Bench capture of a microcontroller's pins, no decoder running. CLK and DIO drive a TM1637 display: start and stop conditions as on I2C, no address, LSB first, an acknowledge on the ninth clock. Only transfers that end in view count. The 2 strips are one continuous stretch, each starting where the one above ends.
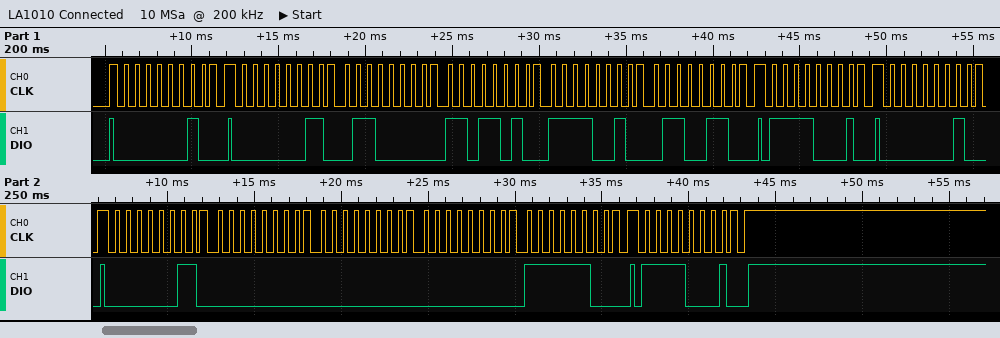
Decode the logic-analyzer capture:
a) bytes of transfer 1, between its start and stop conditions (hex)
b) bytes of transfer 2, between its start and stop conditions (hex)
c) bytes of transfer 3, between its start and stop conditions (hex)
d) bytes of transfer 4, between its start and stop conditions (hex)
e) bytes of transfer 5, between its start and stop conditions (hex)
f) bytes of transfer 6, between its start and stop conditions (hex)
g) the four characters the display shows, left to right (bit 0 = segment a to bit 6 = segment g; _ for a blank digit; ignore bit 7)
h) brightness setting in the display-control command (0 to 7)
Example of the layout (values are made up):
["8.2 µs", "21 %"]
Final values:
["40", "C0 06 5B 4F 66", "8F", "40", "C0 00 00 00 3F", "8F", "___0", "7"]
